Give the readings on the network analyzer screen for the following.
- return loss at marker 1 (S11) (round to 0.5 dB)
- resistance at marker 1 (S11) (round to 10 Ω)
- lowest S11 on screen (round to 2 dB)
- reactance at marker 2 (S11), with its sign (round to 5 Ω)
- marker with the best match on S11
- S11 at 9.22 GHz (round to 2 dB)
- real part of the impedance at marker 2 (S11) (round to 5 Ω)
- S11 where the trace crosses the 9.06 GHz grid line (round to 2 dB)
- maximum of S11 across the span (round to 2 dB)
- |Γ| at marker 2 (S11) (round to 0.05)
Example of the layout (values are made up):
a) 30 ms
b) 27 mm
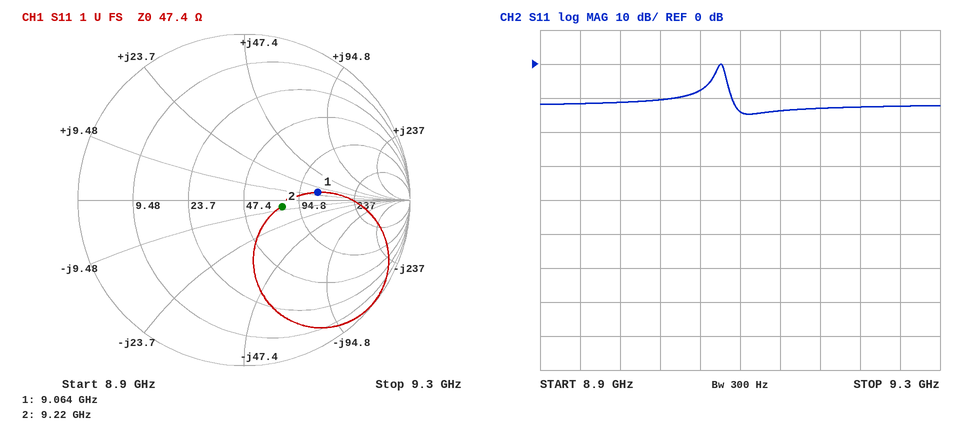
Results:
a) 7.0 dB
b) 120 Ω
c) -14 dB
d) -5 Ω
e) marker 2
f) -12 dB
g) 75 Ω
h) -8 dB
i) 0 dB
j) 0.25
